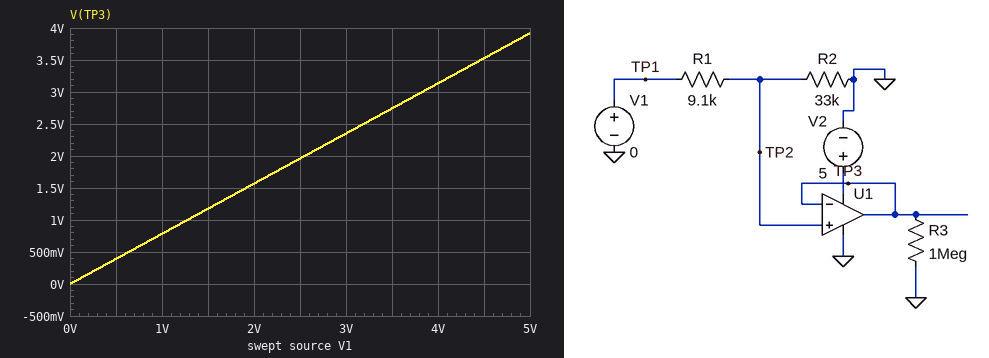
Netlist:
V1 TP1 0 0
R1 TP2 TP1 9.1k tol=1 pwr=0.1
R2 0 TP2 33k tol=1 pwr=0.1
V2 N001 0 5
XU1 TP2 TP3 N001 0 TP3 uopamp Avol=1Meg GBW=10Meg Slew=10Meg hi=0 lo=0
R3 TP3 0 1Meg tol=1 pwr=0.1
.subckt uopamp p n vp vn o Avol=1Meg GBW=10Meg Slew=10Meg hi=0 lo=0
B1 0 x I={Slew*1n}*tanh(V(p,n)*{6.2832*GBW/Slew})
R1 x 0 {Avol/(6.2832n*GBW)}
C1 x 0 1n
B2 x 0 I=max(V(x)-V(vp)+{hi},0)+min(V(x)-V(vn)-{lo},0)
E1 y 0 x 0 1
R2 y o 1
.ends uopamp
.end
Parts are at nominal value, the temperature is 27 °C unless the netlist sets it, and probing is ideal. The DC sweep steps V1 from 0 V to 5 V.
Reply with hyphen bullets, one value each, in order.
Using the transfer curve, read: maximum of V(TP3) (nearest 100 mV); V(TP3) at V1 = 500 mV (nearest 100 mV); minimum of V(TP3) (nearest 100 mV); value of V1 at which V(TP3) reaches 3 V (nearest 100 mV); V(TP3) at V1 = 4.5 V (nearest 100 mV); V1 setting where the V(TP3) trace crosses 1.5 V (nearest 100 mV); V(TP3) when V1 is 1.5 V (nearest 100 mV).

- 3.9 V
- 400 mV
- 0 V
- 3.8 V
- 3.5 V
- 1.9 V
- 1.2 V
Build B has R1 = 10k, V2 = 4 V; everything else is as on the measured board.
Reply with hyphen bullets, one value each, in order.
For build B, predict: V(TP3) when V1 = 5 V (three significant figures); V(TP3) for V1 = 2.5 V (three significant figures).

- 3.84 V
- 1.92 V
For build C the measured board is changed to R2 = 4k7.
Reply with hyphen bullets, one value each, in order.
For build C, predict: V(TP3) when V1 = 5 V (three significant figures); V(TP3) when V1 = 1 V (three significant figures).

- 1.70 V
- 341 mV
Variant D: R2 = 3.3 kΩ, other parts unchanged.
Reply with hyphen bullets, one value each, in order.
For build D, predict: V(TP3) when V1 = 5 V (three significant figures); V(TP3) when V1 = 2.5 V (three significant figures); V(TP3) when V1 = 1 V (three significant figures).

- 1.33 V
- 665 mV
- 266 mV
